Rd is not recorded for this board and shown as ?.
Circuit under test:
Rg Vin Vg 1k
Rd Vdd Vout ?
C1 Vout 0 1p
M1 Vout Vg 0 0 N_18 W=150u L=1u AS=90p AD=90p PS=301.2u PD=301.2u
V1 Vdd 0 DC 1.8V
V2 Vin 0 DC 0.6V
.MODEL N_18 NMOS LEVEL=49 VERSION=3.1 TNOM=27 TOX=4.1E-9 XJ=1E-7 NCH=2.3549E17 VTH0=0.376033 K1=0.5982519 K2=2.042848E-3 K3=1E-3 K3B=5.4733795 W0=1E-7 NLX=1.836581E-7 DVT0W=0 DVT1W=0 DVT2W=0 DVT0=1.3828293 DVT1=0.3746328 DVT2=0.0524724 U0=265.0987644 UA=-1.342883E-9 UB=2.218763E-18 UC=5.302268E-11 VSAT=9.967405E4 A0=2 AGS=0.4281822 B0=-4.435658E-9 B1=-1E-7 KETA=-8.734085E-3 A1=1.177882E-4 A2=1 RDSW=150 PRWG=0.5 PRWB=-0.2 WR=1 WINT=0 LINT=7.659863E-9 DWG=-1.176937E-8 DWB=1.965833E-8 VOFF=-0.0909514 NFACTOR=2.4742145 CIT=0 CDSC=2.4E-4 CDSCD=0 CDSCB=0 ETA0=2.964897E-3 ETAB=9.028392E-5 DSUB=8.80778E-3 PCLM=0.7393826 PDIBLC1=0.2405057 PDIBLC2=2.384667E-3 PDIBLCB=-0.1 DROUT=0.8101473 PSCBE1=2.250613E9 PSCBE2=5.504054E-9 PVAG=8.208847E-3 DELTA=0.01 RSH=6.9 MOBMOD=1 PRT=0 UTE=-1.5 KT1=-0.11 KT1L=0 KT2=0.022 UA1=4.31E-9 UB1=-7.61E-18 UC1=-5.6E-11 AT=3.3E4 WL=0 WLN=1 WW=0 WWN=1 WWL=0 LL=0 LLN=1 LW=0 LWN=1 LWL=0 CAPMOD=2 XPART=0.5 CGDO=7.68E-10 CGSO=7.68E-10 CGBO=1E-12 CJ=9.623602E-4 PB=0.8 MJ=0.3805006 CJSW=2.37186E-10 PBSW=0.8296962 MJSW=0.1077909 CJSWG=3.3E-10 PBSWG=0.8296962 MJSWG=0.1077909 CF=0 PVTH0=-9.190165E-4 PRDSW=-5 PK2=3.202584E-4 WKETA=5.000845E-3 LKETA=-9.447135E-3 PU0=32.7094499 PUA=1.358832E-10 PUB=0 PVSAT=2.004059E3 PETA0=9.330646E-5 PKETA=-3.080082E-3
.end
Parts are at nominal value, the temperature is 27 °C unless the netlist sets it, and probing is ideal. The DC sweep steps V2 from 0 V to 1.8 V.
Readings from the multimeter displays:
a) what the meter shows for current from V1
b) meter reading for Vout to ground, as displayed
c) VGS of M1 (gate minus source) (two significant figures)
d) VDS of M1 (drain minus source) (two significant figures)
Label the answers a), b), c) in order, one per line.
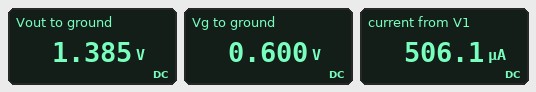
a) 506.1 µA
b) 1.385 V
c) 600 mV
d) 1.4 V
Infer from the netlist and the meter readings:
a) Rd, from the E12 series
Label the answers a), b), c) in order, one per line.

a) 820 Ω
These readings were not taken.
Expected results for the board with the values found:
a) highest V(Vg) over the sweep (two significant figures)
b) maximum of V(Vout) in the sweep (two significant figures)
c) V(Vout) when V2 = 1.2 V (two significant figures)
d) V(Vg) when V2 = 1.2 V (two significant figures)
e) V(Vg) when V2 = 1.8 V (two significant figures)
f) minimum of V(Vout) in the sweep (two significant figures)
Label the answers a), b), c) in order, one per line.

a) 1.8 V
b) 1.8 V
c) 100 mV
d) 1.2 V
e) 1.8 V
f) 76 mV
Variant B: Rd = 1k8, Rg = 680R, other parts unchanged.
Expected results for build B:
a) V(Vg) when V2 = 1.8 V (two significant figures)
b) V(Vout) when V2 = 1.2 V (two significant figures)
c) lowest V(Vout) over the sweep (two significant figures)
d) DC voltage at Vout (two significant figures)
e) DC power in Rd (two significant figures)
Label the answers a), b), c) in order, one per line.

a) 1.8 V
b) 47 mV
c) 35 mV
d) 930 mV
e) 420 µW
